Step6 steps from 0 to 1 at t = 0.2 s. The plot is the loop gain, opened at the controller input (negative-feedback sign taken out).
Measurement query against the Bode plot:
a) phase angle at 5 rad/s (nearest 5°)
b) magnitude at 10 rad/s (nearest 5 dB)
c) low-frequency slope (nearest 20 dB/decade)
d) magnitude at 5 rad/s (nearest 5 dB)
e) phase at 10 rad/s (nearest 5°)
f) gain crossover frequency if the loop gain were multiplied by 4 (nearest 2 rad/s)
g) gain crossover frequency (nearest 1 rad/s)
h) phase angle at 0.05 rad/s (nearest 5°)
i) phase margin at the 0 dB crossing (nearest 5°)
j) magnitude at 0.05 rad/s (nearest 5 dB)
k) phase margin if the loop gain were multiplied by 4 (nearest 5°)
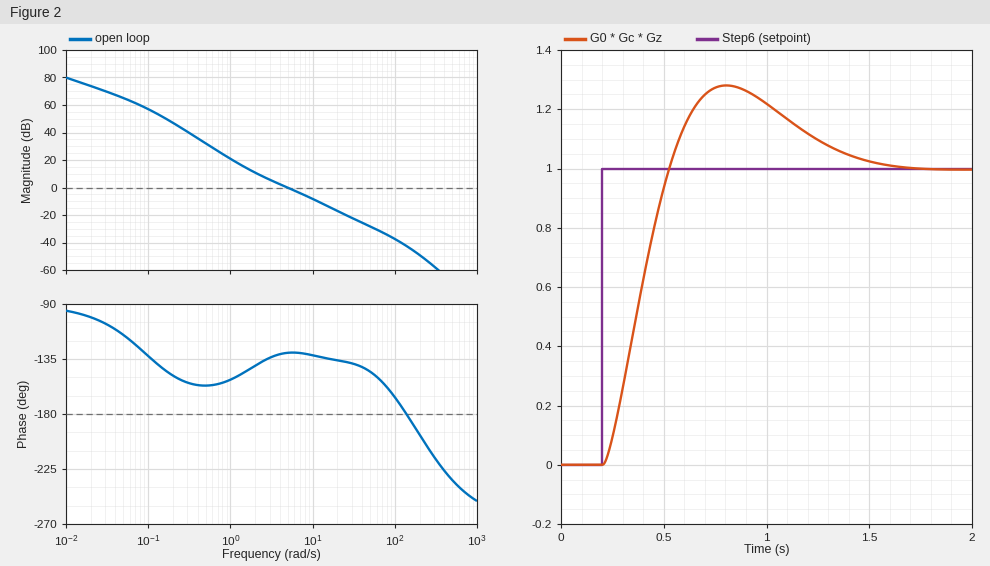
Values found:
-130°
-10 dB
-20 dB/decade
0 dB
-130°
14 rad/s
5 rad/s
-115°
50°
65 dB
45°
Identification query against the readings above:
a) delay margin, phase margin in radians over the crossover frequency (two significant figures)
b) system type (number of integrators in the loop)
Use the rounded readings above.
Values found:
0.17 s
1
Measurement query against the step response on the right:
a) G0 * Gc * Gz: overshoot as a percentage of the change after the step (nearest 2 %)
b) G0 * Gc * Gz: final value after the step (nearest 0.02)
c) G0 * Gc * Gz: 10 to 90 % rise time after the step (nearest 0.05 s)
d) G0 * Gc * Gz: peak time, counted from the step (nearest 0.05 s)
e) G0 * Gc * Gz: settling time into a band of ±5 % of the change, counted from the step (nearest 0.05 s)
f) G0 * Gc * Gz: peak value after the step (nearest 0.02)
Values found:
28 %
1.00
0.25 s
0.60 s
1.20 s
1.28
